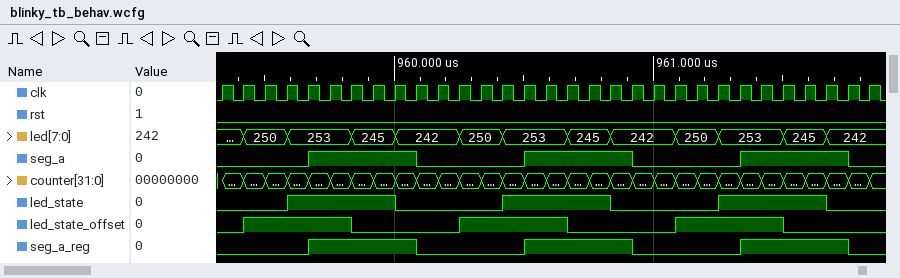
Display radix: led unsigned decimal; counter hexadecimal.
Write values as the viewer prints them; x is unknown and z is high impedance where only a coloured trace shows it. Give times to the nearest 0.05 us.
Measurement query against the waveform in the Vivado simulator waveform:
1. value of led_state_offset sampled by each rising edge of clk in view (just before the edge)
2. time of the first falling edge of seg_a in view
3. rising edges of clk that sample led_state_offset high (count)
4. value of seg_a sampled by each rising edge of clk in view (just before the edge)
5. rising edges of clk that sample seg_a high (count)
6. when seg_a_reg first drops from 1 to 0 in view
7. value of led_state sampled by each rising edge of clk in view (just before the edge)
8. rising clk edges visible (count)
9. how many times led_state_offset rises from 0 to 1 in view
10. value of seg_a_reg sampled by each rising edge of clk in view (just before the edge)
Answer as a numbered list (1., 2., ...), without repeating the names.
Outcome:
1. 0 0 1 1 1 1 1 0 0 0 0 0 1 1 1 1 1 0 0 0 0 0 1 1 1 1 1 0 0 0 0
2. 960.1 us
3. 15
4. 0 0 0 0 0 1 1 1 1 1 0 0 0 0 0 1 1 1 1 1 0 0 0 0 0 1 1 1 1 1 0
5. 15
6. 960.1 us
7. 0 0 0 0 1 1 1 1 1 0 0 0 0 0 1 1 1 1 1 0 0 0 0 0 1 1 1 1 1 0 0
8. 31
9. 3
10. 0 0 0 0 0 1 1 1 1 1 0 0 0 0 0 1 1 1 1 1 0 0 0 0 0 1 1 1 1 1 0
